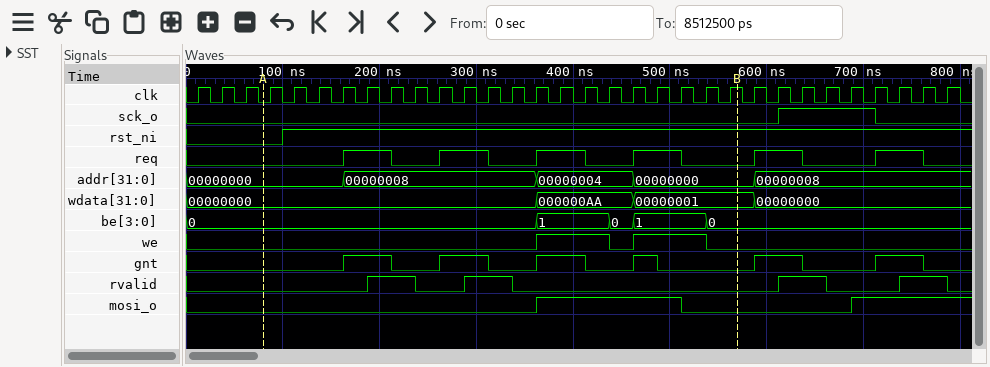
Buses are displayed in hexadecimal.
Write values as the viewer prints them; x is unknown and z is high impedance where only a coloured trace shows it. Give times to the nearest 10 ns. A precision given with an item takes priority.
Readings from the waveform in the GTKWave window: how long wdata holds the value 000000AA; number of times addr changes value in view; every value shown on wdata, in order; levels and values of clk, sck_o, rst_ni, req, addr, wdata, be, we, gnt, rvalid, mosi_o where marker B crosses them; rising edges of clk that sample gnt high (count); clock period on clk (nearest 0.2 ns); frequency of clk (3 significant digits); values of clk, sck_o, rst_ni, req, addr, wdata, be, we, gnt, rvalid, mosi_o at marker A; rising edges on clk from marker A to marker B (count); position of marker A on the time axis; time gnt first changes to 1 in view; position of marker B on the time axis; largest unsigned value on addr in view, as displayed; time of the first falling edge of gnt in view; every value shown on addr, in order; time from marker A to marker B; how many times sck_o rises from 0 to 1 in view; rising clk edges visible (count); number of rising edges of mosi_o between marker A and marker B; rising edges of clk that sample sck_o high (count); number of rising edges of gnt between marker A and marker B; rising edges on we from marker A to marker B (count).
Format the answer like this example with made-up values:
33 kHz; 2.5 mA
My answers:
100 ns; 4; 00000000, 000000AA, 00000001, 00000000; clk=1, sck_o=0, rst_ni=1, req=0, addr=00000000, wdata=00000001, be=0, we=0, gnt=0, rvalid=0, mosi_o=0; 11; 25 ns; 40.0 MHz; clk=0, sck_o=0, rst_ni=0, req=0, addr=00000000, wdata=00000000, be=0, we=0, gnt=0, rvalid=0, mosi_o=0; 20; 80 ns; 160 ns; 570 ns; 00000008; 210 ns; 00000000, 00000008, 00000004, 00000000, 00000008; 490 ns; 1; 32; 1; 4; 4; 2
